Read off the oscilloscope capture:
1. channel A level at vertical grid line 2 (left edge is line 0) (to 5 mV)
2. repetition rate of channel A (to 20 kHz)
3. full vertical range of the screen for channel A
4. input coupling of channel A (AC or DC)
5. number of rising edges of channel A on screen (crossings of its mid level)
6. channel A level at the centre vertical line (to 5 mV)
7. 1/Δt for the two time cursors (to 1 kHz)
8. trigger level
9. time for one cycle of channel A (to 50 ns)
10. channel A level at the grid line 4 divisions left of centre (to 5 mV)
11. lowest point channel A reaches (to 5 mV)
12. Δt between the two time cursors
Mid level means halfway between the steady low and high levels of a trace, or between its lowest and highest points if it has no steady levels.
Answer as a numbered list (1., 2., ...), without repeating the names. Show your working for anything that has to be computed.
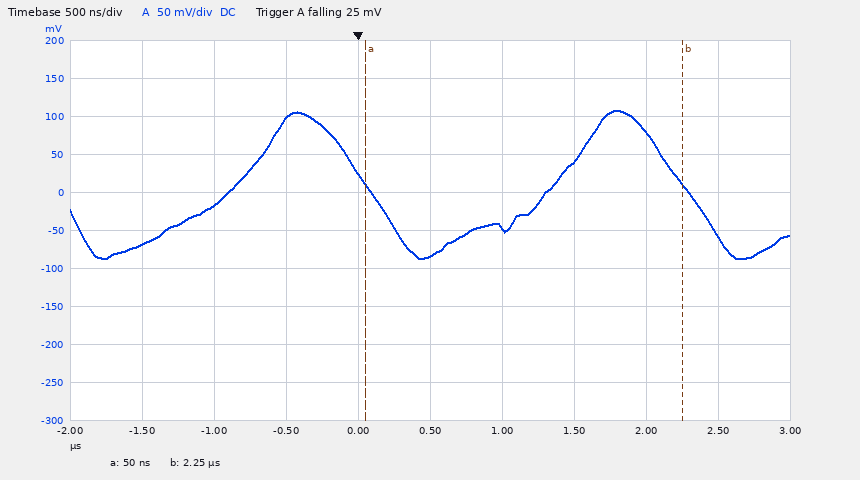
1. -15 mV
2. 1 / 2.20 µs ≈ 455 kHz, so 460 kHz to the nearest 20 kHz
3. 500 mV
4. DC
5. 2
6. -85 mV
7. 1 / 2.20 µs ≈ 455 kHz
8. 25 mV
9. 2.20 µs
10. -70 mV
11. -85 mV
12. 2.25 µs − (50 ns) = 2.20 µs
